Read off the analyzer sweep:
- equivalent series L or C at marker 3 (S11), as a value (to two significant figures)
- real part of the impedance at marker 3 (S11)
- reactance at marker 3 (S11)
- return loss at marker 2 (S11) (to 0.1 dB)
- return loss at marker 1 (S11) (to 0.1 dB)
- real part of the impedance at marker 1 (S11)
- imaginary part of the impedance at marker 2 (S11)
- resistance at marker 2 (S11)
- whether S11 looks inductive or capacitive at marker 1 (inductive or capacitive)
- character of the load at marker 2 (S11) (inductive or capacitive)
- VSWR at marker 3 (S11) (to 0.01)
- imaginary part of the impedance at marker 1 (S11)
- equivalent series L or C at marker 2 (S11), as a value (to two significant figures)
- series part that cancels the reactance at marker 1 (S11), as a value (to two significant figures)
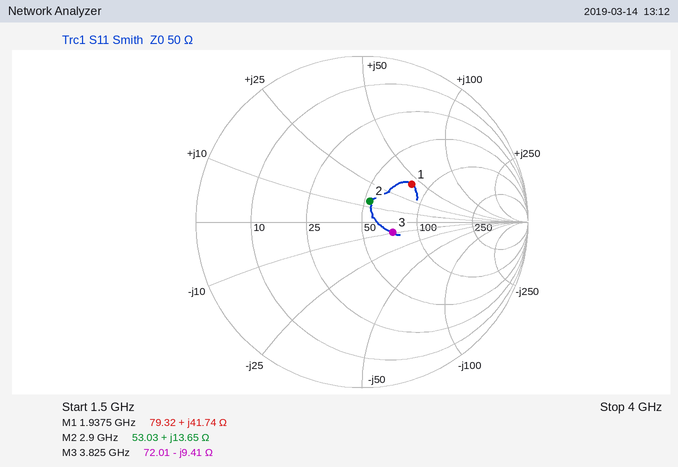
4.4 pF
72.01 Ω
-9.41 Ω
17.4 dB
8.5 dB
79.32 Ω
+13.65 Ω
53.03 Ω
inductive
inductive
1.49
+41.74 Ω
750 pH
2.0 pF
